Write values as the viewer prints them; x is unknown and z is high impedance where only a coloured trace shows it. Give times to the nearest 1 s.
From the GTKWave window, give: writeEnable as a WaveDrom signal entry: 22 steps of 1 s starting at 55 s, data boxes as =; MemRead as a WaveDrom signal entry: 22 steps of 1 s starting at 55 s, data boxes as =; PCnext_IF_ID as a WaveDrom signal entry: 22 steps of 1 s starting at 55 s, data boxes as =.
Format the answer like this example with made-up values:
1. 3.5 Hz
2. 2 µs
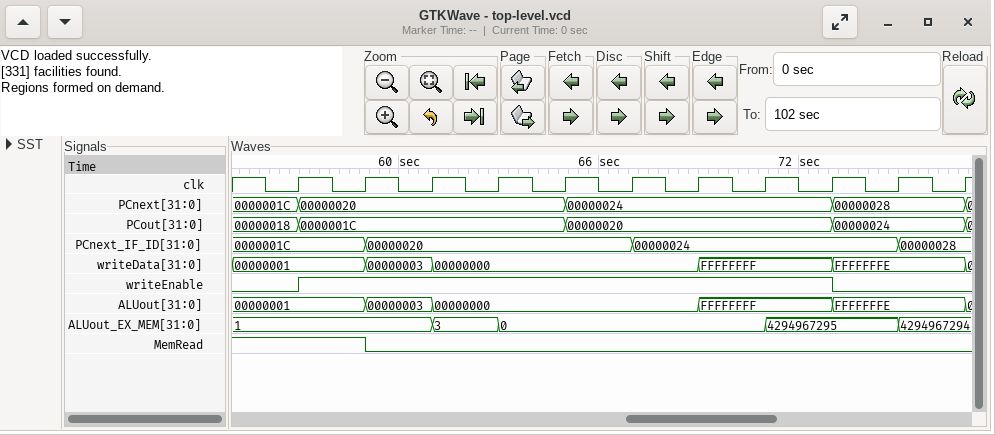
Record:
1. {name: 'writeEnable', wave: '0.1...............0...'}
2. {name: 'MemRead', wave: '1...0.................'}
3. {name: 'PCnext_IF_ID', wave: '=...=.......=.......=.', data: '0000001C 00000020 00000024 00000028'}
